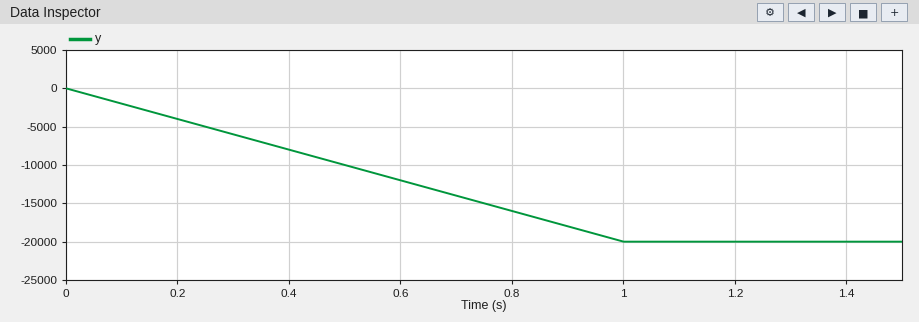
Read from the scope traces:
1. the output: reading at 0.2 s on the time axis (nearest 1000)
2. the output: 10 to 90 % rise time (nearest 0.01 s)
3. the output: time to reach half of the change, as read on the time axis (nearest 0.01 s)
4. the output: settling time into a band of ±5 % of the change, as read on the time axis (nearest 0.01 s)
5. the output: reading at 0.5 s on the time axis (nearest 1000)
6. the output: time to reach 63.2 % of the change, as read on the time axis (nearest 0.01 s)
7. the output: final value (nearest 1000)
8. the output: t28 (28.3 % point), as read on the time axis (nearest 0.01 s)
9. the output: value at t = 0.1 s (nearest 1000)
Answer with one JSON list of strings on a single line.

["-4000", "0.80 s", "0.50 s", "0.95 s", "-10000", "0.63 s", "-20000", "0.28 s", "-2000"]
